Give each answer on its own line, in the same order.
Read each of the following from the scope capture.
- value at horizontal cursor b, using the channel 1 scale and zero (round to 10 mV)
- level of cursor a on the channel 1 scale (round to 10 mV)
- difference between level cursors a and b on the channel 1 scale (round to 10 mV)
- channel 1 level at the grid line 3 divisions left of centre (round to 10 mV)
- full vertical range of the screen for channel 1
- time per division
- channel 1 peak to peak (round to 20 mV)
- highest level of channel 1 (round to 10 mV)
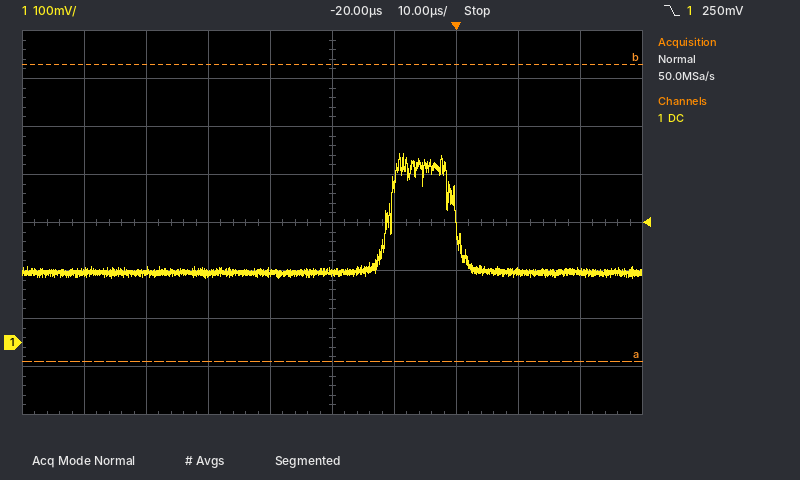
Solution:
580 mV
-40 mV
620 mV
150 mV
800 mV
10 µs
260 mV
390 mV
